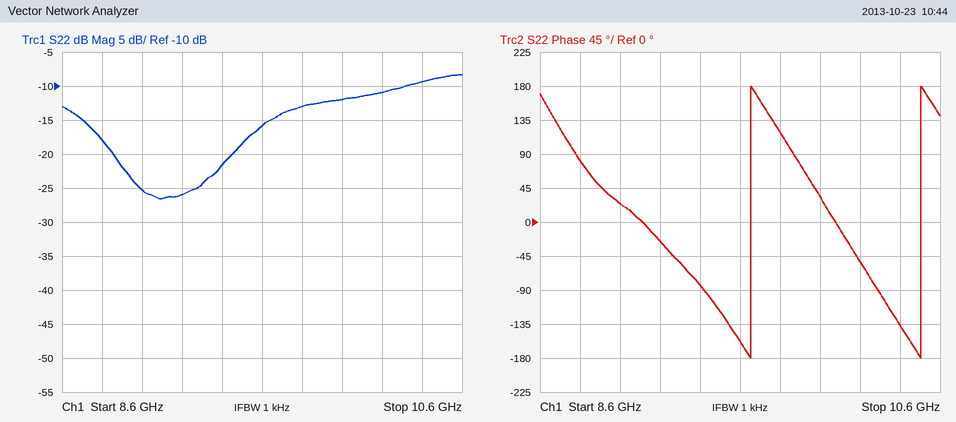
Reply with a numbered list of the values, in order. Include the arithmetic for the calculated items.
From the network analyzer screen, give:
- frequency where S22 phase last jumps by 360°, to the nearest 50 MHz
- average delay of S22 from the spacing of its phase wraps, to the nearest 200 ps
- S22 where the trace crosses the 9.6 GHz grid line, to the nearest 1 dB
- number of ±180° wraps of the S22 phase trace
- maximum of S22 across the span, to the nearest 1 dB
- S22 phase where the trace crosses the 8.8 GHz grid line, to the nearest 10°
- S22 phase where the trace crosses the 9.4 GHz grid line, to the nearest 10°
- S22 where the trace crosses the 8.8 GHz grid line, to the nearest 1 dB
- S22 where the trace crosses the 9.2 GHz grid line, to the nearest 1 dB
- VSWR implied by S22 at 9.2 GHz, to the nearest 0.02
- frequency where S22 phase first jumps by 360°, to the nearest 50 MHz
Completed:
1. 10.50 GHz
2. 1 cycle / (10.50 GHz − 9.65 GHz) ≈ 1.2 ns
3. -16 dB
4. 2
5. -8 dB
6. 80°
7. -80°
8. -18 dB
9. -26 dB
10. |Γ| = 10^(-26/20) = 0.0501; VSWR = (1 + 0.0501)/(1 − 0.0501) ≈ 1.11, so 1.10 to the nearest 0.02
11. 9.65 GHz
